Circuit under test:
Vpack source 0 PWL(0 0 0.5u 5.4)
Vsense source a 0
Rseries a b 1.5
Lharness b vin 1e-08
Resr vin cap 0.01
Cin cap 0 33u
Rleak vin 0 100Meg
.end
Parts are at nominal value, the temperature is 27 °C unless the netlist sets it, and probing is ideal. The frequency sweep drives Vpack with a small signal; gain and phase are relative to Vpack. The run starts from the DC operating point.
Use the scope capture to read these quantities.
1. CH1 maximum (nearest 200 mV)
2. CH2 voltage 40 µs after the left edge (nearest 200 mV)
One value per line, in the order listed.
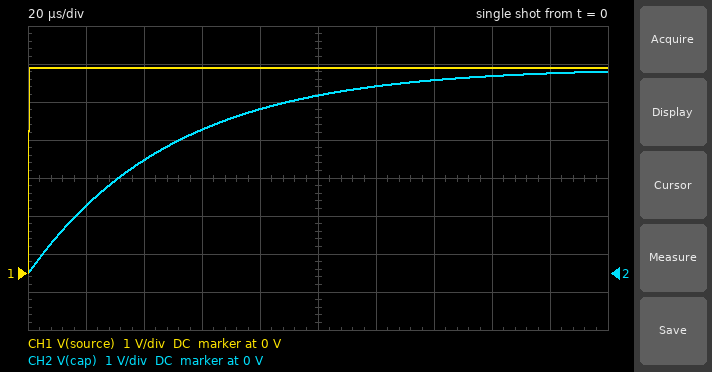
5.4 V
3.0 V
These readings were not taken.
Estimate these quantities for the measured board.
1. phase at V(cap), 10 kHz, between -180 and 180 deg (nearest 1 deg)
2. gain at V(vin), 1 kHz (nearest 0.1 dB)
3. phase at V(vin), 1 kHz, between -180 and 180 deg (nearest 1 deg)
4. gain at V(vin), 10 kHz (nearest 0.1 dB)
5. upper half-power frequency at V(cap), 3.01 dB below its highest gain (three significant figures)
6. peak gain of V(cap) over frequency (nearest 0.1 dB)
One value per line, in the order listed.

-72 deg
-0.4 dB
-17 deg
-10.3 dB
3.19 kHz
0 dB
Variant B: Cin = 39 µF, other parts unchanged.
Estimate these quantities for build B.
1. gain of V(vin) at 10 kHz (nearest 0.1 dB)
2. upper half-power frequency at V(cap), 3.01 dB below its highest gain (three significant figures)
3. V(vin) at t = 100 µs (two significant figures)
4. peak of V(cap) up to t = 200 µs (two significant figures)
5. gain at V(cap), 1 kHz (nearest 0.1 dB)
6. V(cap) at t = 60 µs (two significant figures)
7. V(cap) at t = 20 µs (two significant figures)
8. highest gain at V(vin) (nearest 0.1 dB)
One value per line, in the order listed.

-11.7 dB
2.70 kHz
4.4 V
5.2 V
-0.6 dB
3.4 V
1.5 V
0 dB
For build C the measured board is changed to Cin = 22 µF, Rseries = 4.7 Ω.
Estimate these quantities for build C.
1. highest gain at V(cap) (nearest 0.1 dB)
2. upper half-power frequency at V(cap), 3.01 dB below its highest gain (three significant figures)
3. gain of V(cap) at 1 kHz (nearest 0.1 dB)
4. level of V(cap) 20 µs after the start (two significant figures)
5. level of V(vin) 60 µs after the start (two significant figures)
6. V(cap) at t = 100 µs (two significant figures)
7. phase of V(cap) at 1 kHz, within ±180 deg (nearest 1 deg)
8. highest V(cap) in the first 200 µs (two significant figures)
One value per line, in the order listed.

0 dB
1.54 kHz
-1.5 dB
940 mV
2.4 V
3.3 V
-33 deg
4.6 V
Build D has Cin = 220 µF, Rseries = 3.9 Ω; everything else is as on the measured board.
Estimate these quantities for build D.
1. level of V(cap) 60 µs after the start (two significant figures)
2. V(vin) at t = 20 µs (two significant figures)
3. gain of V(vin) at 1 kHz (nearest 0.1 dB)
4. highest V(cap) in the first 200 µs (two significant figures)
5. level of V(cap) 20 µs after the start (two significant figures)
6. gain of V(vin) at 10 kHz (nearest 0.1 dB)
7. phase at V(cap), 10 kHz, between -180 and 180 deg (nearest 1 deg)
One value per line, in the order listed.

360 mV
140 mV
-14.8 dB
1.1 V
120 mV
-34.6 dB
-89 deg
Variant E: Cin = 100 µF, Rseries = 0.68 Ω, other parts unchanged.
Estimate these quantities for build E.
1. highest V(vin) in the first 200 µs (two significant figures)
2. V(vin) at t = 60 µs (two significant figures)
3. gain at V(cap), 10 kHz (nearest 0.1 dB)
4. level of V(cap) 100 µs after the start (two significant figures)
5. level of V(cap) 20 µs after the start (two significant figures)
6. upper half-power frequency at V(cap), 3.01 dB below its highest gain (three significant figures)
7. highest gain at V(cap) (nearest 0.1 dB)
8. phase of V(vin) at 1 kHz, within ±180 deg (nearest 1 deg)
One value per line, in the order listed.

5.1 V
3.2 V
-13.0 dB
4.1 V
1.3 V
2.31 kHz
0 dB
-23 deg
